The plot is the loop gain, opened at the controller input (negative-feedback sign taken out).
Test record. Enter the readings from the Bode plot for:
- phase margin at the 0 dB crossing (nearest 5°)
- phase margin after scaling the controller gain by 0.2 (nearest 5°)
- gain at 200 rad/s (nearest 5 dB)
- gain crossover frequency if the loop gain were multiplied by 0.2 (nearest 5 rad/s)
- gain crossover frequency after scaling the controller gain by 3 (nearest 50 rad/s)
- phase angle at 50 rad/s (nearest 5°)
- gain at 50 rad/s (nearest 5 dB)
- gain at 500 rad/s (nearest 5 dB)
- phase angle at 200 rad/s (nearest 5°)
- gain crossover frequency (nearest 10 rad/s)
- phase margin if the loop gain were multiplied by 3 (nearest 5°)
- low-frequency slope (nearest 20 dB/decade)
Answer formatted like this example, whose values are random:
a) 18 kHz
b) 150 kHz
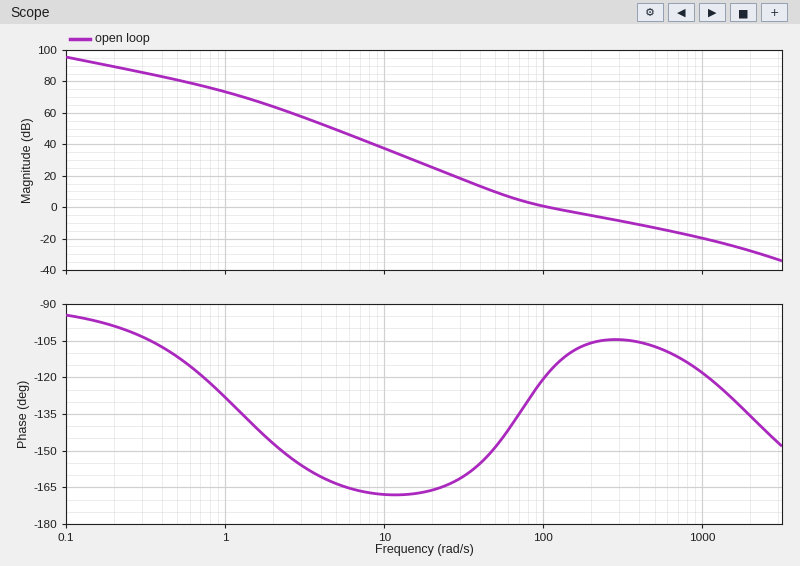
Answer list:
a) 60°
b) 25°
c) -5 dB
d) 40 rad/s
e) 350 rad/s
f) -150°
g) 10 dB
h) -15 dB
i) -105°
j) 110 rad/s
k) 75°
l) -20 dB/decade
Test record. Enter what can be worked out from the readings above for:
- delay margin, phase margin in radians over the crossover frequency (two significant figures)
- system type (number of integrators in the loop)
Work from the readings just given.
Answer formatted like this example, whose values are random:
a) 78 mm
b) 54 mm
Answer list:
a) 0.0095 s
b) 1
